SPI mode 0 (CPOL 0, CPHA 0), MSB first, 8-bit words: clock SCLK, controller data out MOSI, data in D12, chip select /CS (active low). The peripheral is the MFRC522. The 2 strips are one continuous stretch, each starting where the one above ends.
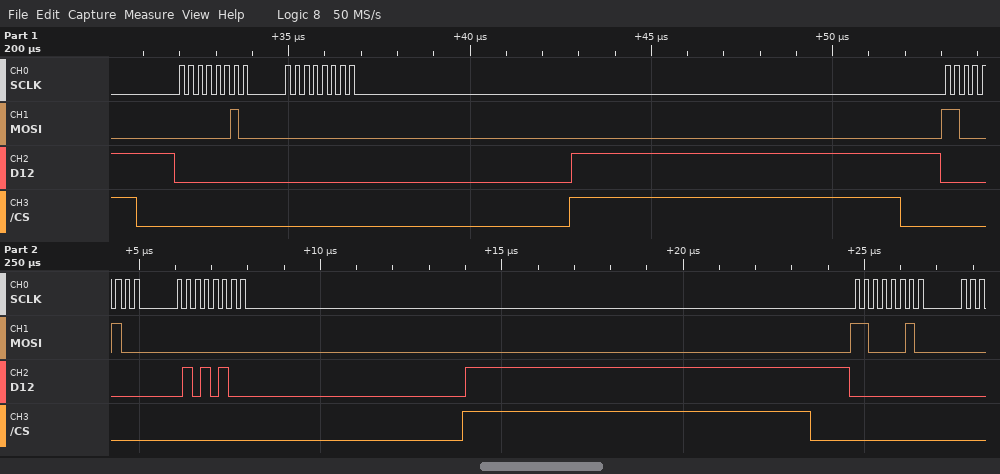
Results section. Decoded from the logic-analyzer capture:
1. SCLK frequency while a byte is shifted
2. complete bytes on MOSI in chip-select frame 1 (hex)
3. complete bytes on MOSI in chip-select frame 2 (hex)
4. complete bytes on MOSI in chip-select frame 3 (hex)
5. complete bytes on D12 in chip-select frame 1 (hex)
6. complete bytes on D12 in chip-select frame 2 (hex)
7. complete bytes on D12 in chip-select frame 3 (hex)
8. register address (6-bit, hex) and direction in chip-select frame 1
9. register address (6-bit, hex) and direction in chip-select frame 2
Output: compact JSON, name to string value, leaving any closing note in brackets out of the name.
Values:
{"SCLK frequency while a byte is shifted": "4 MHz", "complete bytes on MOSI in chip-select frame 1": "02 00", "complete bytes on MOSI in chip-select frame 2": "C4 00", "complete bytes on MOSI in chip-select frame 3": "C2", "complete bytes on D12 in chip-select frame 1": "00 00", "complete bytes on D12 in chip-select frame 2": "00 54", "complete bytes on D12 in chip-select frame 3": "00", "register address (6-bit, hex) and direction in chip-select frame 1": "0x01 write", "register address (6-bit, hex) and direction in chip-select frame 2": "0x22 read"}
